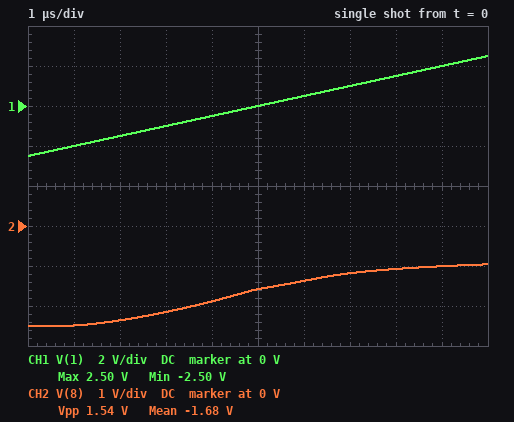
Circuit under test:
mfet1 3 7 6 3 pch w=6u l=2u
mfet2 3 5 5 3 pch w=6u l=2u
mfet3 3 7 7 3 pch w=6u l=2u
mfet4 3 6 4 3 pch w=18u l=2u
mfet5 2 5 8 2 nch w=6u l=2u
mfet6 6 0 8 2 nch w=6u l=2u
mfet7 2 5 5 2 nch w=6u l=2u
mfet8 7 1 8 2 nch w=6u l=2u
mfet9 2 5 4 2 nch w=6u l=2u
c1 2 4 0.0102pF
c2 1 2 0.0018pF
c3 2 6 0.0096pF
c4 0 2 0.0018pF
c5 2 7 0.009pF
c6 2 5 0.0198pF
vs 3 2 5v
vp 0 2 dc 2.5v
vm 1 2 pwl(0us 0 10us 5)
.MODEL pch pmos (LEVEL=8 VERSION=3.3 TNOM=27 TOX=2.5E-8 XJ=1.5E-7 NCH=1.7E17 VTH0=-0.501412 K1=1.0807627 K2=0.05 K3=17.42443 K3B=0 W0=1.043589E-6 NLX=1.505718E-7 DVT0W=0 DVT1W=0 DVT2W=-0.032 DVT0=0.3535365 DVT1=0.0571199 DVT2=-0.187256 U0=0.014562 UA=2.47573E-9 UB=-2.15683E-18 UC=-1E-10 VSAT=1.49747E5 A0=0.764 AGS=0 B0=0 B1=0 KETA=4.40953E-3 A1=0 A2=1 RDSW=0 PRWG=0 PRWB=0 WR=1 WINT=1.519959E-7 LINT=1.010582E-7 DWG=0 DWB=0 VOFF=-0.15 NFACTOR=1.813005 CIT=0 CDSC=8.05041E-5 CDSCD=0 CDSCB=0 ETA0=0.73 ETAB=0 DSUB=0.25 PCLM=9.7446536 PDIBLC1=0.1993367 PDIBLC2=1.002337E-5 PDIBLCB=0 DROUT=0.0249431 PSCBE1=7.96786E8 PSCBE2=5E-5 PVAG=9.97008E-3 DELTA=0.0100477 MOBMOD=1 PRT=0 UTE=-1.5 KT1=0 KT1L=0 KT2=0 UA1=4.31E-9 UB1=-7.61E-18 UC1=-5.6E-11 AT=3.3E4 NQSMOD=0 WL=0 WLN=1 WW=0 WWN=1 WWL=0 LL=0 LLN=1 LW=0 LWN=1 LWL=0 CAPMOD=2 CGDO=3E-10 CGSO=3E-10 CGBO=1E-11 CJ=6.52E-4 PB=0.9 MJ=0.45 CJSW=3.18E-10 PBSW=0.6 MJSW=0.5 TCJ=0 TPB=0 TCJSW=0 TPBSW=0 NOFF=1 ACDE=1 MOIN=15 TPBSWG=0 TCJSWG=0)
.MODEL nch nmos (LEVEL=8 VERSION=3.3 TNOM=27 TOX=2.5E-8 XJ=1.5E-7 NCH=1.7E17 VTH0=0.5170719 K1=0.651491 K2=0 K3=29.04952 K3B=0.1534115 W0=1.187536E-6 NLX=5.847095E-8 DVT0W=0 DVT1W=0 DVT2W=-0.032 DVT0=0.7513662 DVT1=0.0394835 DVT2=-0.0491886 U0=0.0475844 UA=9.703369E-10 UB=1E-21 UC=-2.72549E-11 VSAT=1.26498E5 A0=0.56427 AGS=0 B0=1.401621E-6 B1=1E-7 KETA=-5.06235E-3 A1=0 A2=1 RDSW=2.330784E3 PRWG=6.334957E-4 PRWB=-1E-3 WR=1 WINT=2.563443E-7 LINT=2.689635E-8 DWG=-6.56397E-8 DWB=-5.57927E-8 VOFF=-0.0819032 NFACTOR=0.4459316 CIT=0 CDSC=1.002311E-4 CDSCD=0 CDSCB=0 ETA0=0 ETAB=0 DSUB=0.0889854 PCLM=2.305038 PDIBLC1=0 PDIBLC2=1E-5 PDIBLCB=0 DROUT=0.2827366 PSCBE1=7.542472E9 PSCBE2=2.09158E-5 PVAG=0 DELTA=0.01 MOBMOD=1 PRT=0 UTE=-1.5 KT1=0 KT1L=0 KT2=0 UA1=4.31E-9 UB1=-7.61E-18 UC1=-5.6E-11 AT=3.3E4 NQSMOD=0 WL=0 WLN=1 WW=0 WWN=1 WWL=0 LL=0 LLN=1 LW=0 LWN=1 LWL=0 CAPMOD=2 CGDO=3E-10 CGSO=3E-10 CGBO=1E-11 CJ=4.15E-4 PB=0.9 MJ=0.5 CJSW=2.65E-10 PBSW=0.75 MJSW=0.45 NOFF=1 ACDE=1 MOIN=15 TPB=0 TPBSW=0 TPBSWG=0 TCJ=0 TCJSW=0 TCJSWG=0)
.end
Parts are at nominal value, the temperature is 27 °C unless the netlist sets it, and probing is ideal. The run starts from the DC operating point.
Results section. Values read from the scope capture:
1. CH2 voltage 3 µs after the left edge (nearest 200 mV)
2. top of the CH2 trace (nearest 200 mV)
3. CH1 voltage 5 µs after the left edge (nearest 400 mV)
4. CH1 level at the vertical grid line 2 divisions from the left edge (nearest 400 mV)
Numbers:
-2.2 V
-1.0 V
0 V
-1.6 V
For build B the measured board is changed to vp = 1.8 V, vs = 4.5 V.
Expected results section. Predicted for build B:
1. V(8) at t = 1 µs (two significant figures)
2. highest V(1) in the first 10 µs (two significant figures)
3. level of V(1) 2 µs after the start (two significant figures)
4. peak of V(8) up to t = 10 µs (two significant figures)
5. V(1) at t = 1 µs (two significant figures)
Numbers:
-1.8 V
3.2 V
-800 mV
-370 mV
-1.3 V
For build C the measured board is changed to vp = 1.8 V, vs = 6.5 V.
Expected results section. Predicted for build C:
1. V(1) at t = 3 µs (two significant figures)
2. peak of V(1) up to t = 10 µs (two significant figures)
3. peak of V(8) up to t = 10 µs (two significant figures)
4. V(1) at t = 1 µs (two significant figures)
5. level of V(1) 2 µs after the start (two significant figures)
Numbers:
-300 mV
3.2 V
-130 mV
-1.3 V
-800 mV
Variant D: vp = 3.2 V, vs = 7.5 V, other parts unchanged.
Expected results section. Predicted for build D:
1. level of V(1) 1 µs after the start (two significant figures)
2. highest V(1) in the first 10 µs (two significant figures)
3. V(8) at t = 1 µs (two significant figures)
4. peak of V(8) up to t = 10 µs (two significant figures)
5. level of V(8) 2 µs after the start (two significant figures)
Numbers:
-2.7 V
1.8 V
-3.2 V
-1.4 V
-3.1 V
